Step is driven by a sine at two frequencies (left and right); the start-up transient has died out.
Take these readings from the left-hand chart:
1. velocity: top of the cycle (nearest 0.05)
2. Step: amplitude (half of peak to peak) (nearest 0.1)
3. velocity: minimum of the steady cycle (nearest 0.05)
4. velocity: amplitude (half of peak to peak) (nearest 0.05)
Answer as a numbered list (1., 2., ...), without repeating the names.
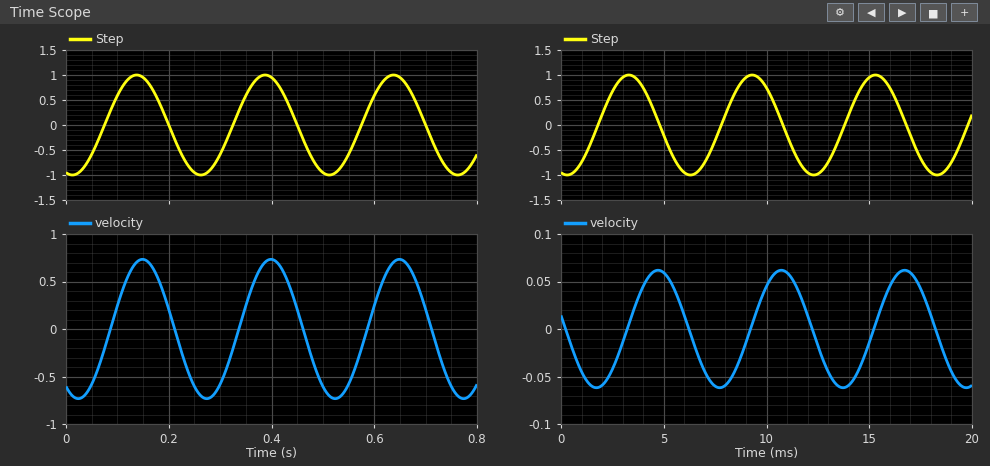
1. 0.75
2. 1.0
3. -0.75
4. 0.75
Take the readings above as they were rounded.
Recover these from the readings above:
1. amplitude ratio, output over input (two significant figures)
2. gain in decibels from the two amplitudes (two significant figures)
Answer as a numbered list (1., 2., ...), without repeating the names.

1. 0.75
2. -2.5 dB
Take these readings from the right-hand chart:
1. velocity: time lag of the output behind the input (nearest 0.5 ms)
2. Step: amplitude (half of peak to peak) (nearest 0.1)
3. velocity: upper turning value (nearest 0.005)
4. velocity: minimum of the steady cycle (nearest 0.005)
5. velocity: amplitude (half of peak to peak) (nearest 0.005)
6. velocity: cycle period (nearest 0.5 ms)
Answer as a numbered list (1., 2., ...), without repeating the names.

1. 1.5 ms
2. 1.0
3. 0.060
4. -0.060
5. 0.060
6. 6.0 ms
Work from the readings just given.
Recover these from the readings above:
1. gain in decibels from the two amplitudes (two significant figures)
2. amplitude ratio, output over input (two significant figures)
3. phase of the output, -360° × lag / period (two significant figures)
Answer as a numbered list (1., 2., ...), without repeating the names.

1. -24 dB
2. 0.060
3. -90°
